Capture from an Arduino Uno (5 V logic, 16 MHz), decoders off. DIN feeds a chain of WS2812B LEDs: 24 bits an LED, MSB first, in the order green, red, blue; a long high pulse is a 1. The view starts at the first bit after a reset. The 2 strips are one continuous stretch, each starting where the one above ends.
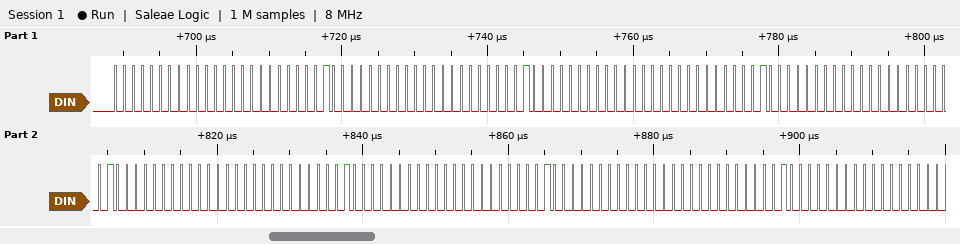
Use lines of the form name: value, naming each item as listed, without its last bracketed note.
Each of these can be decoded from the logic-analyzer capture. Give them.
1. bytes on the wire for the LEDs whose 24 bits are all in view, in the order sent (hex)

bytes on the wire for the LEDs whose 24 bits are all in view, in the order sent: 00 00 01 00 00 04 00 00 01 00 00 04 00 00 01 00 00 04 00 00 01
